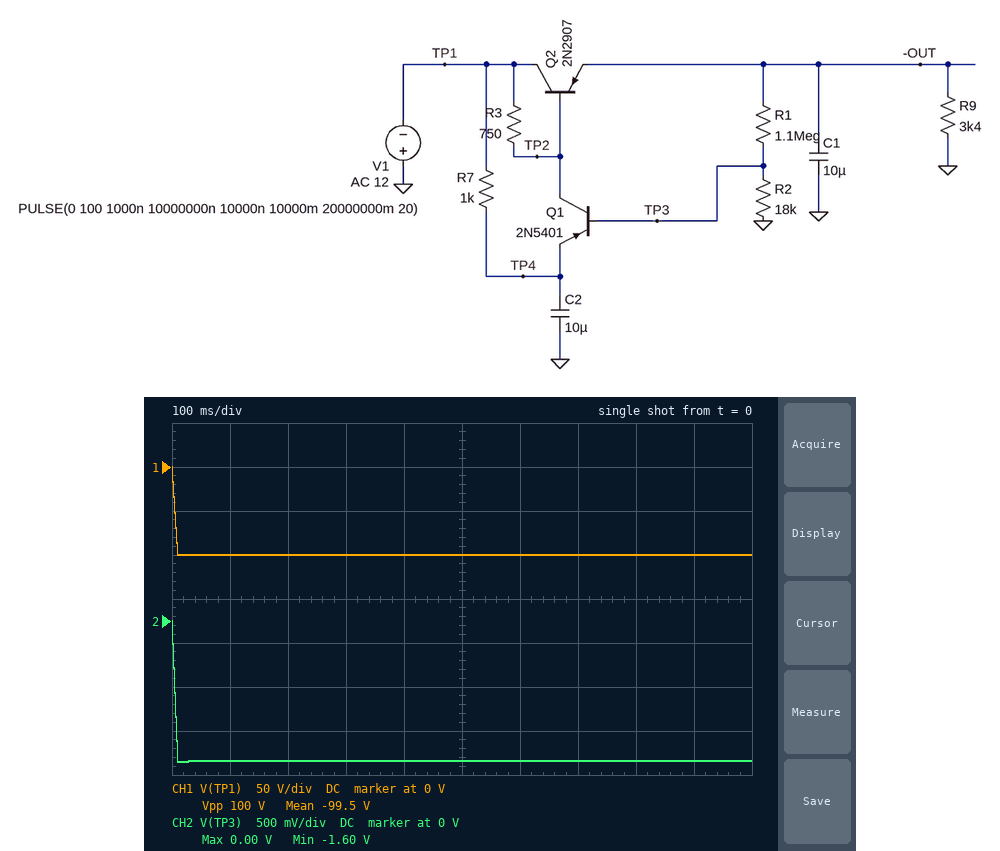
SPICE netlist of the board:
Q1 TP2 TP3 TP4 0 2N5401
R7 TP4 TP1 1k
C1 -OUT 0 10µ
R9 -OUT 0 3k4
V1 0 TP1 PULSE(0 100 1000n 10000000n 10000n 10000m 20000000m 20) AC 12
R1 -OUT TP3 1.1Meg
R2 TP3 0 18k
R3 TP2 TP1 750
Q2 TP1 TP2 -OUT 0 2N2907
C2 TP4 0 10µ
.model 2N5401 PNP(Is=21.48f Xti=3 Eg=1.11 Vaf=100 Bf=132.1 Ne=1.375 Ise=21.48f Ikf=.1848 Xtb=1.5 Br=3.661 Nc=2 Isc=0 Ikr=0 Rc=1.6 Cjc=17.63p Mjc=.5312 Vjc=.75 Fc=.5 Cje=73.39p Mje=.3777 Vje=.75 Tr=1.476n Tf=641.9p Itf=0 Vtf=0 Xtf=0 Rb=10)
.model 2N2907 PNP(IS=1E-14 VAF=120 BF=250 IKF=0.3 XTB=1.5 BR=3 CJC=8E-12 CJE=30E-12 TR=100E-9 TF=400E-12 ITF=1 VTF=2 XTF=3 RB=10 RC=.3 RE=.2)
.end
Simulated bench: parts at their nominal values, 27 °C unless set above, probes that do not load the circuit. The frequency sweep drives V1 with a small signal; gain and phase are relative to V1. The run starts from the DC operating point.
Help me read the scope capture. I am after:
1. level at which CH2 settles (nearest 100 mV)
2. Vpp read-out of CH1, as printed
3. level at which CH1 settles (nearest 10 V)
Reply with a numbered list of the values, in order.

1. -1.6 V
2. 100 V
3. -100 V
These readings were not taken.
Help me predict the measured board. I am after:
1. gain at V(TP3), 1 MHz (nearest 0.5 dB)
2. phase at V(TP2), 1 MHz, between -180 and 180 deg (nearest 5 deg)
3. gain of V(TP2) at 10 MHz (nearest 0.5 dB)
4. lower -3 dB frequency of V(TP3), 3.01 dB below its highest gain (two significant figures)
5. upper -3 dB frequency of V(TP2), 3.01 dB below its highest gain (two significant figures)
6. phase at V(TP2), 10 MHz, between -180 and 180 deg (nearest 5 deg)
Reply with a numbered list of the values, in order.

1. -14.5 dB
2. 170 deg
3. -8.0 dB
4. 94 kHz
5. 4.1 MHz
6. 135 deg
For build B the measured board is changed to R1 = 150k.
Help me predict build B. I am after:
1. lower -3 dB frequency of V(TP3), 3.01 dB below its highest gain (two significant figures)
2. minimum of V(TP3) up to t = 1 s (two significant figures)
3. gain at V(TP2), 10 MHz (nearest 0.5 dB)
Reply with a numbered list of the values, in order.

1. 100 kHz
2. -11 V
3. -8.0 dB
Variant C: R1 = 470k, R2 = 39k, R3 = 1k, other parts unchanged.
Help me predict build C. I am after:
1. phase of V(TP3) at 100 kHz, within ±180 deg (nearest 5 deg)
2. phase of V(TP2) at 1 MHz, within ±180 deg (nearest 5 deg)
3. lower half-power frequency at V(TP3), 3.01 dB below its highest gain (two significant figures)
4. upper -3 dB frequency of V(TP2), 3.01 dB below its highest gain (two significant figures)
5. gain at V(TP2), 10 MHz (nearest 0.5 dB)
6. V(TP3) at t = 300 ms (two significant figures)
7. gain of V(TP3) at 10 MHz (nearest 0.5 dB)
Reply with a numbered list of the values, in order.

1. -155 deg
2. 165 deg
3. 47 kHz
4. 3.1 MHz
5. -9.5 dB
6. -7.6 V
7. -24.0 dB
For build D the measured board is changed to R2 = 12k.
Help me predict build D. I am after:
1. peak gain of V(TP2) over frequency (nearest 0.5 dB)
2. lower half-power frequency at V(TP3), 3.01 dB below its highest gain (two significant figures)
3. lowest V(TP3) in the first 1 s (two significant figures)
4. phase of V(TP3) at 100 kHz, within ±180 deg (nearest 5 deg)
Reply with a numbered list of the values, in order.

1. 0 dB
2. 140 kHz
3. -1.1 V
4. -125 deg
